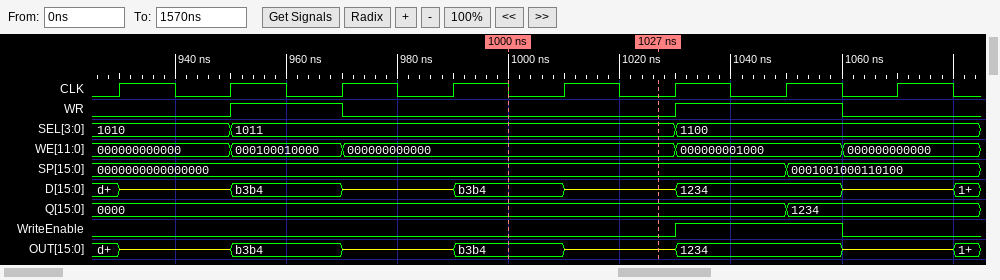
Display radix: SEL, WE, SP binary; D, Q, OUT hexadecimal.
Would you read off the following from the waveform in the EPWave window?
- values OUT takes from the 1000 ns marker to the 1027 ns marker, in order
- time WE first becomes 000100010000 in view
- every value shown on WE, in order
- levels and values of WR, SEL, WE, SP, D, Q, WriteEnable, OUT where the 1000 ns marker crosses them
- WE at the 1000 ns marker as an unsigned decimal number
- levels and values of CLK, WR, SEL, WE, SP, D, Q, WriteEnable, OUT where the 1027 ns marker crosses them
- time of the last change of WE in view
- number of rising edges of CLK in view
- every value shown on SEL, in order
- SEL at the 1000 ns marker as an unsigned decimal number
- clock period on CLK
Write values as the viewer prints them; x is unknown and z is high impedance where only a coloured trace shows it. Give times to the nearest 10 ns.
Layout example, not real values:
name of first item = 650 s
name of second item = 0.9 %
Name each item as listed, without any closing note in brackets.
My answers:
values OUT takes from the 1000 ns marker to the 1027 ns marker, in order = b3b4, z
time WE first becomes 000100010000 in view = 950 ns
every value shown on WE, in order = 000000000000, 000100010000, 000000000000, 000000001000, 000000000000
levels and values of WR, SEL, WE, SP, D, Q, WriteEnable, OUT where the 1000 ns marker crosses them = WR=0, SEL=1011, WE=000000000000, SP=0000000000000000, D=b3b4, Q=0000, WriteEnable=0, OUT=b3b4
WE at the 1000 ns marker as an unsigned decimal number = 0
levels and values of CLK, WR, SEL, WE, SP, D, Q, WriteEnable, OUT where the 1027 ns marker crosses them = CLK=0, WR=0, SEL=1011, WE=000000000000, SP=0000000000000000, D=z, Q=0000, WriteEnable=0, OUT=z
time of the last change of WE in view = 1060 ns
number of rising edges of CLK in view = 8
every value shown on SEL, in order = 1010, 1011, 1100
SEL at the 1000 ns marker as an unsigned decimal number = 11
clock period on CLK = 20 ns
